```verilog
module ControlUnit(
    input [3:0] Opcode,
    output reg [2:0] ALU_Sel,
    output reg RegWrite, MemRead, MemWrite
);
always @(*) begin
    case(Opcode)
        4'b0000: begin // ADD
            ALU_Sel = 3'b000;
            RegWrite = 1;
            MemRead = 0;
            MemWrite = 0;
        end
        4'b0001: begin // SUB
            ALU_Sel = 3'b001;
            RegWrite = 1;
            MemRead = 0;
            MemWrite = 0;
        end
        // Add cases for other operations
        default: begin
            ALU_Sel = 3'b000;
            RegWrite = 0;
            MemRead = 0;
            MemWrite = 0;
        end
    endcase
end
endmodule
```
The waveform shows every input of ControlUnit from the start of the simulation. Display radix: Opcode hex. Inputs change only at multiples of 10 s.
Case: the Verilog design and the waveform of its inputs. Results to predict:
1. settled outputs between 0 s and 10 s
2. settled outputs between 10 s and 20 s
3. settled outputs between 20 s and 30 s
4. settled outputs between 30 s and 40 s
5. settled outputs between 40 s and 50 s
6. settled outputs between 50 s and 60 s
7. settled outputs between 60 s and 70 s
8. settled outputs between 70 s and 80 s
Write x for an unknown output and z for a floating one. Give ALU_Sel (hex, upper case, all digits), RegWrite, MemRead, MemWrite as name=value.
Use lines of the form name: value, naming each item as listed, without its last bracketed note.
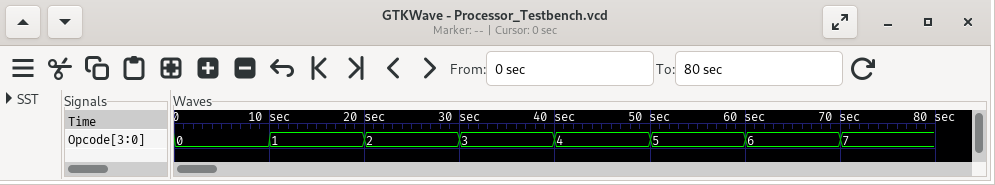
settled outputs between 0 s and 10 s: ALU_Sel=0, RegWrite=1, MemRead=0, MemWrite=0
settled outputs between 10 s and 20 s: ALU_Sel=1, RegWrite=1, MemRead=0, MemWrite=0
settled outputs between 20 s and 30 s: ALU_Sel=0, RegWrite=0, MemRead=0, MemWrite=0
settled outputs between 30 s and 40 s: ALU_Sel=0, RegWrite=0, MemRead=0, MemWrite=0
settled outputs between 40 s and 50 s: ALU_Sel=0, RegWrite=0, MemRead=0, MemWrite=0
settled outputs between 50 s and 60 s: ALU_Sel=0, RegWrite=0, MemRead=0, MemWrite=0
settled outputs between 60 s and 70 s: ALU_Sel=0, RegWrite=0, MemRead=0, MemWrite=0
settled outputs between 70 s and 80 s: ALU_Sel=0, RegWrite=0, MemRead=0, MemWrite=0
